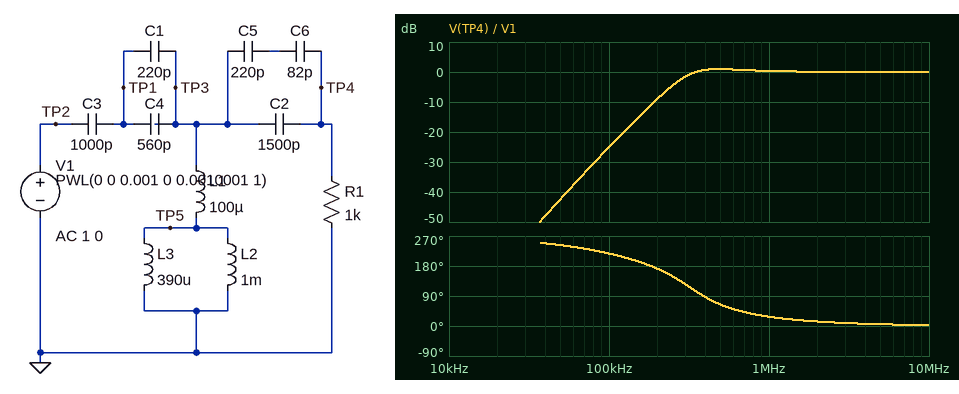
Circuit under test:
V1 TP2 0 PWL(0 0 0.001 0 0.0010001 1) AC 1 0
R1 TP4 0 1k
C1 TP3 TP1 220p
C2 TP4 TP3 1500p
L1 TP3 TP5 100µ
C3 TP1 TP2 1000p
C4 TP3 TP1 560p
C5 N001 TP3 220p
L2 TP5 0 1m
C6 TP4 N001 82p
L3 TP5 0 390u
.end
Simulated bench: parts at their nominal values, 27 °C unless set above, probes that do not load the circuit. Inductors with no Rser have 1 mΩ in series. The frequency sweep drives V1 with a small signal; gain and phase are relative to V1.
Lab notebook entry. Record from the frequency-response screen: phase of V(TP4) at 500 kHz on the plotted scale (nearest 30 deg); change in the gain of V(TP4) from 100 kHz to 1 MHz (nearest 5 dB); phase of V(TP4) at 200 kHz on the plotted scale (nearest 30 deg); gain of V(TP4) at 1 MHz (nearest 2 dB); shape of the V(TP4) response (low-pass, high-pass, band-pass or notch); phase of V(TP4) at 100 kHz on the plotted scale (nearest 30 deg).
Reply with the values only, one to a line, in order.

60 deg
25 dB
180 deg
0 dB
high-pass
210 deg
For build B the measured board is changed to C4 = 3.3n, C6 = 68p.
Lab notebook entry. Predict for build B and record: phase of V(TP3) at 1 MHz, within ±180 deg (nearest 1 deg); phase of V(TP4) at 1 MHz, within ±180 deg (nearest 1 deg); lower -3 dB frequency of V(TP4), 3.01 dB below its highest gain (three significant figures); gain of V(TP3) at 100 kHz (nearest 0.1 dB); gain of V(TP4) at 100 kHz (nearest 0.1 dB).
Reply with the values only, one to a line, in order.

12 deg
18 deg
217 kHz
-16.4 dB
-19.5 dB
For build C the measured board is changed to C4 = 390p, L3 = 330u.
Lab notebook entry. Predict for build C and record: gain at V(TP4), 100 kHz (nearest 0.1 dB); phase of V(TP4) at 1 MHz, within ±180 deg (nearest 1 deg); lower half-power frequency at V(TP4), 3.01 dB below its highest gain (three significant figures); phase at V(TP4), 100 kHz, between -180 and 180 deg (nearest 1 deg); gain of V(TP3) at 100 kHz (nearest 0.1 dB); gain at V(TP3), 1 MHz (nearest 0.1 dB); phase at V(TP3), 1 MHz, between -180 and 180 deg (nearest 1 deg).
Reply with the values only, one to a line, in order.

-27.3 dB
32 deg
331 kHz
-142 deg
-24.2 dB
0.5 dB
26 deg
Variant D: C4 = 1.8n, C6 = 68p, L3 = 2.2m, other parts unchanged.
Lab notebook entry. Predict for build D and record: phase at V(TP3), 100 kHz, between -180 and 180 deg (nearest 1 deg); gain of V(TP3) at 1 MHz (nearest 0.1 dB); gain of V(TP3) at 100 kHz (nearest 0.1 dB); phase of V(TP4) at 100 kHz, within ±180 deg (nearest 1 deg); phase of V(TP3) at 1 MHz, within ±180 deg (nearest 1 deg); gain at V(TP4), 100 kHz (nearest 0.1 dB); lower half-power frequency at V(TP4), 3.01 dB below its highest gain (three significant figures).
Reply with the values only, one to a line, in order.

156 deg
0 dB
-9.1 dB
-158 deg
14 deg
-12.3 dB
149 kHz
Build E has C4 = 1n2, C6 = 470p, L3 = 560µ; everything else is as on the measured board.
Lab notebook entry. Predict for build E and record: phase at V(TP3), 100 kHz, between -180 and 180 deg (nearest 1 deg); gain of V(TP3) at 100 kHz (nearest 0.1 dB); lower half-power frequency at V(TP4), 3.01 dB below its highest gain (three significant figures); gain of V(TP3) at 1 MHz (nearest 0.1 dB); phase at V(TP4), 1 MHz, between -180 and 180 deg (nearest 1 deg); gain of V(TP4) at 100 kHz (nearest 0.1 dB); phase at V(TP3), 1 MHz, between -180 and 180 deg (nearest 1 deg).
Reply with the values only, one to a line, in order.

169 deg
-17.1 dB
222 kHz
0.3 dB
22 deg
-20.0 dB
16 deg
